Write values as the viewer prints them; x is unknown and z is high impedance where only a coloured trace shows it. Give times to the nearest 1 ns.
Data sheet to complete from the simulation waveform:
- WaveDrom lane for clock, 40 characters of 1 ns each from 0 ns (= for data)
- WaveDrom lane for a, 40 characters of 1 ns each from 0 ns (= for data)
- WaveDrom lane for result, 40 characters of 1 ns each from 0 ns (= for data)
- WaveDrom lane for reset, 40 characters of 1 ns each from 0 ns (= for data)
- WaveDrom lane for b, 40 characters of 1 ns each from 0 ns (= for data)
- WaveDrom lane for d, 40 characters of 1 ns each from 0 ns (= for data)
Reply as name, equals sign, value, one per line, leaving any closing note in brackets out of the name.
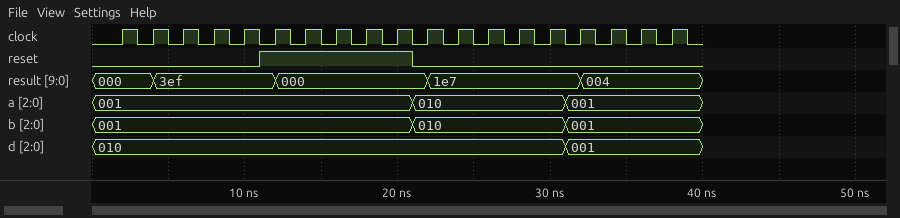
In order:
WaveDrom lane for clock, 40 characters of 1 ns each from 0 ns = {name: 'clock', wave: '0.10101010101010101010101010101010101010'}
WaveDrom lane for a, 40 characters of 1 ns each from 0 ns = {name: 'a', wave: '=....................=.........=........', data: '001 010 001'}
WaveDrom lane for result, 40 characters of 1 ns each from 0 ns = {name: 'result', wave: '=...=.......=.........=.........=.......', data: '000 3ef 000 1e7 004'}
WaveDrom lane for reset, 40 characters of 1 ns each from 0 ns = {name: 'reset', wave: '0..........1.........0..................'}
WaveDrom lane for b, 40 characters of 1 ns each from 0 ns = {name: 'b', wave: '=....................=.........=........', data: '001 010 001'}
WaveDrom lane for d, 40 characters of 1 ns each from 0 ns = {name: 'd', wave: '=..............................=........', data: '010 001'}
